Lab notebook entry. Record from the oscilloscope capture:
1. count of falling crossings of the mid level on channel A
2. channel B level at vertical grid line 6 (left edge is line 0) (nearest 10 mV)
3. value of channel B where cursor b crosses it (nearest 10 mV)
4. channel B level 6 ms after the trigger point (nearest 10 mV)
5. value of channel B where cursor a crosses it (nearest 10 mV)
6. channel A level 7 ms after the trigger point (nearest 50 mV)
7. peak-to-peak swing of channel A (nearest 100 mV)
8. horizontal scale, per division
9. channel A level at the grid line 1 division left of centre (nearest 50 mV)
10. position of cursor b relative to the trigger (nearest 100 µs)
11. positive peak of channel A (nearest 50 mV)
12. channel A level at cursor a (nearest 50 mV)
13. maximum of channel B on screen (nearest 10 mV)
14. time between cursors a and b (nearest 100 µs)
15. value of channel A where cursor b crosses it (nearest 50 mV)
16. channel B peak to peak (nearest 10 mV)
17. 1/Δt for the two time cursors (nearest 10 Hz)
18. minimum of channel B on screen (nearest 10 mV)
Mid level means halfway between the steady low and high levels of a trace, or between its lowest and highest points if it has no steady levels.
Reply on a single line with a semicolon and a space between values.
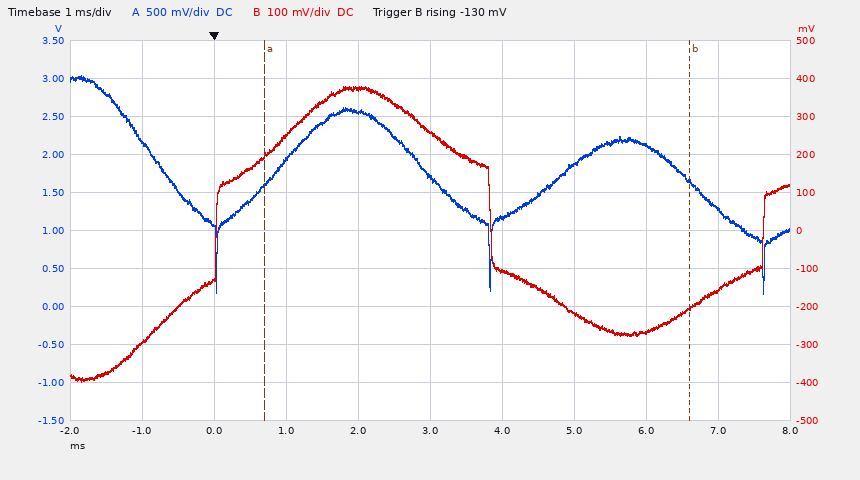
3; -110 mV; -200 mV; -270 mV; 200 mV; 1.30 V; 2.90 V; 1 ms; 2.55 V; +6.6 ms; 3.05 V; 1.60 V; 380 mV; 5.9 ms; 1.65 V; 780 mV; 170 Hz; -400 mV
